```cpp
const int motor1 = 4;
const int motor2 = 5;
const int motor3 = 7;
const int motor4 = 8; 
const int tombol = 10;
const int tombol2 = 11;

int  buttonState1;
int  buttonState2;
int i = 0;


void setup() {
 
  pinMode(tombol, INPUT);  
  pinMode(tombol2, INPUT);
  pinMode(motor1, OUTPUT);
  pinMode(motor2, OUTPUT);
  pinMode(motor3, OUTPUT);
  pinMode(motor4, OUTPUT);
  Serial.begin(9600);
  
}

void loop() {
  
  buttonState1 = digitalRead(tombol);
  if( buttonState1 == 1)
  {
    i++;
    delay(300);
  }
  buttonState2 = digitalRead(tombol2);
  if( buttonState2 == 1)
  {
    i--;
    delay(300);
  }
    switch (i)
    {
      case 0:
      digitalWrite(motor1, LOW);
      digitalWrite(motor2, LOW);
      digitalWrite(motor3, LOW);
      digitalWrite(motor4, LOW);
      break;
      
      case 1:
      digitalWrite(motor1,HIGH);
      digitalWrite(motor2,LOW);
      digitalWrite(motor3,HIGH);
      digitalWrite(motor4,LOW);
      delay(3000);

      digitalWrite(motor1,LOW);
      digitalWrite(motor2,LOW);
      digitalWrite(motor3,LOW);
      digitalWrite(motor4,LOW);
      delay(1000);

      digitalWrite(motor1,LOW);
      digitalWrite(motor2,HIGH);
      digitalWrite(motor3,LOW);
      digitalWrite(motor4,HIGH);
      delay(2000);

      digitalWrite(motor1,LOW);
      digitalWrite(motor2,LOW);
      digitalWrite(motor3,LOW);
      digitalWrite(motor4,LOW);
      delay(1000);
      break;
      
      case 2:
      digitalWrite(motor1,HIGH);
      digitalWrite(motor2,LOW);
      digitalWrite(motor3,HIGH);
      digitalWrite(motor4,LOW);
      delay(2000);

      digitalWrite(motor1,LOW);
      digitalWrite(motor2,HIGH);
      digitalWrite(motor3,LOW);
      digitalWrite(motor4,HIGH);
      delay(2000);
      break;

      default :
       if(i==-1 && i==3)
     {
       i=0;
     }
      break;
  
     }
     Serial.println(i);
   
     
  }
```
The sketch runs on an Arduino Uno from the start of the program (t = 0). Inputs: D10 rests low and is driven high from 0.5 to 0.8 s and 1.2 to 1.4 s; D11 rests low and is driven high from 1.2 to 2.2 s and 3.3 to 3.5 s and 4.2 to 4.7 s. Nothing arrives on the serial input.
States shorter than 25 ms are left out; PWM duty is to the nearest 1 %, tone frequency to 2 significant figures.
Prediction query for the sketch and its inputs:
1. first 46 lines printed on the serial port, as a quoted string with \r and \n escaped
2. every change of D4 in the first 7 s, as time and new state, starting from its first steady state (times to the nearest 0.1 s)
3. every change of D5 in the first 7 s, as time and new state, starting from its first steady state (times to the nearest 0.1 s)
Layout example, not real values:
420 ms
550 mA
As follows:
"0\r\n0\r\n0\r\n0\r\n0\r\n0\r\n0\r\n0\r\n0\r\n0\r\n0\r\n0\r\n0\r\n0\r\n0\r\n0\r\n0\r\n0\r\n0\r\n0\r\n0\r\n0\r\n0\r\n0\r\n0\r\n0\r\n0\r\n0\r\n0\r\n0\r\n0\r\n0\r\n0\r\n0\r\n0\r\n0\r\n0\r\n0\r\n0\r\n0\r\n0\r\n0\r\n0\r\n0\r\n0\r\n0\r\n"
0 s low; 0.8 s high; 3.8 s low
0 s low; 4.8 s high; 6.8 s low
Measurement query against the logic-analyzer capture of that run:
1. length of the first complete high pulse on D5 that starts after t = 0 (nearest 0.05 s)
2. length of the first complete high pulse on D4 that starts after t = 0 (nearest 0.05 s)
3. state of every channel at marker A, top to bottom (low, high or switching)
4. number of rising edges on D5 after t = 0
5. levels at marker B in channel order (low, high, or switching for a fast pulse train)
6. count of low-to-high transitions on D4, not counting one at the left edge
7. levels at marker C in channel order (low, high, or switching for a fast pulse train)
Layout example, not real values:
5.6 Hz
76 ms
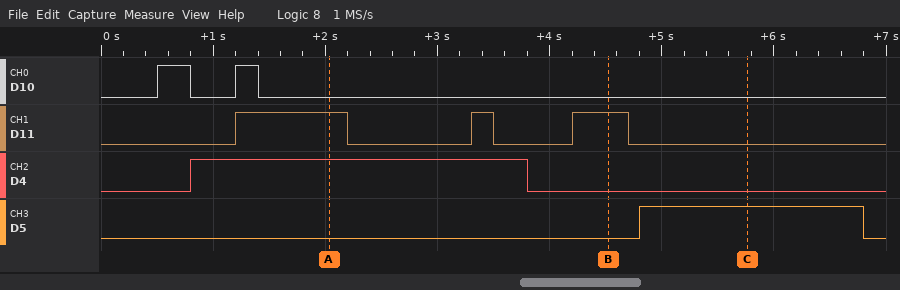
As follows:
2.00 s
3.00 s
D10 low, D11 high, D4 high, D5 low
1
D10 low, D11 high, D4 low, D5 low
1
D10 low, D11 low, D4 low, D5 high
